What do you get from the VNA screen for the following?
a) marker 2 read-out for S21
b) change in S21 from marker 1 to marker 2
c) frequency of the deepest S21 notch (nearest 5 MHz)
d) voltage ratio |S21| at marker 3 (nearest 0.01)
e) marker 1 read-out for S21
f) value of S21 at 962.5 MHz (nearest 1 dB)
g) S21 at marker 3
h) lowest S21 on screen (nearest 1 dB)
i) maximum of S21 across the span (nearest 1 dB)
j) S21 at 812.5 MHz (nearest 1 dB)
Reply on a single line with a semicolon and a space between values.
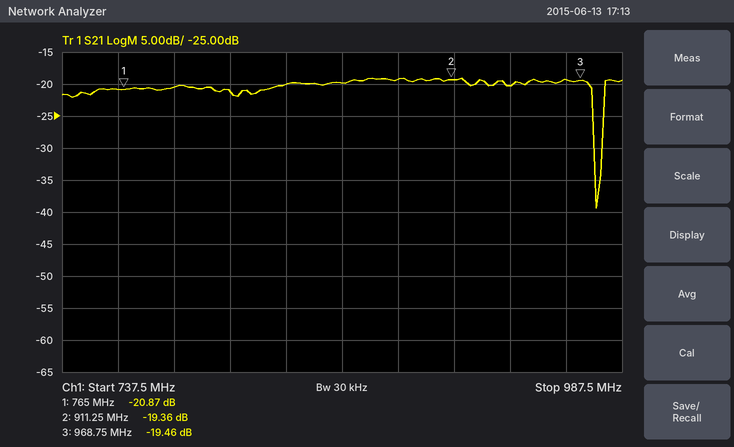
-19.36 dB; 1.51 dB; 975 MHz; 0.11; -20.87 dB; -19 dB; -19.46 dB; -39 dB; -19 dB; -21 dB
